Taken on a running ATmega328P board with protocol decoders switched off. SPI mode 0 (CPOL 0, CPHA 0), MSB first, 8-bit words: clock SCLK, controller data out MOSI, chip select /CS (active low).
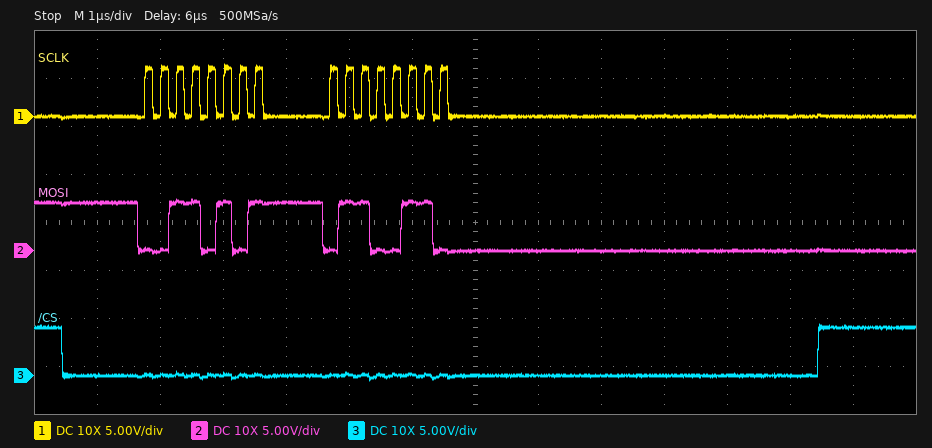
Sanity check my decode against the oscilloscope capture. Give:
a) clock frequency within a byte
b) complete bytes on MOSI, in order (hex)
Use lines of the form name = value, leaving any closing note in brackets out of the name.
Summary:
clock frequency within a byte = 4 MHz
complete bytes on MOSI, in order = 35 66
